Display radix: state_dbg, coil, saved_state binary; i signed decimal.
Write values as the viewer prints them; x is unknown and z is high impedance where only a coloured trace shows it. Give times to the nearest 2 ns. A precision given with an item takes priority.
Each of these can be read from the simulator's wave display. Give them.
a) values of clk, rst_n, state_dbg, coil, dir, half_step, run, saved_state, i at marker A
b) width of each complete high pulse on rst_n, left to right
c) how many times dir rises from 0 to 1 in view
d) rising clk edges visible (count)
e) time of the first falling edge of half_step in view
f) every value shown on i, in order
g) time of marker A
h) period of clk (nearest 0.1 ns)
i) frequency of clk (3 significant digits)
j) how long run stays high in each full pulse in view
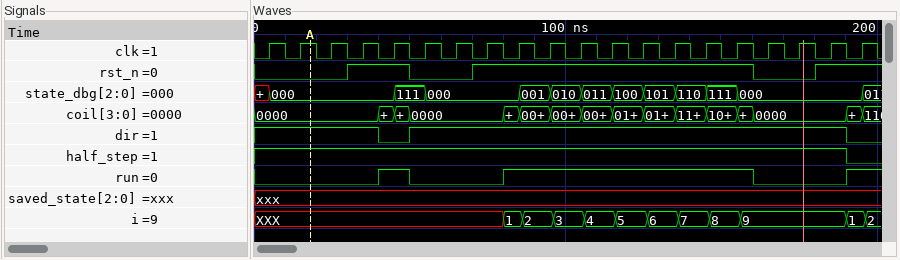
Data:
clk=1, rst_n=0, state_dbg=000, coil=0000, dir=1, half_step=1, run=0, saved_state=xxx, i=XXX
20 ns, 90 ns
1
20
190 ns
XXX, 1, 2, 3, 4, 5, 6, 7, 8, 9, 1, 2
18 ns
10 ns
100 MHz
10 ns, 80 ns
